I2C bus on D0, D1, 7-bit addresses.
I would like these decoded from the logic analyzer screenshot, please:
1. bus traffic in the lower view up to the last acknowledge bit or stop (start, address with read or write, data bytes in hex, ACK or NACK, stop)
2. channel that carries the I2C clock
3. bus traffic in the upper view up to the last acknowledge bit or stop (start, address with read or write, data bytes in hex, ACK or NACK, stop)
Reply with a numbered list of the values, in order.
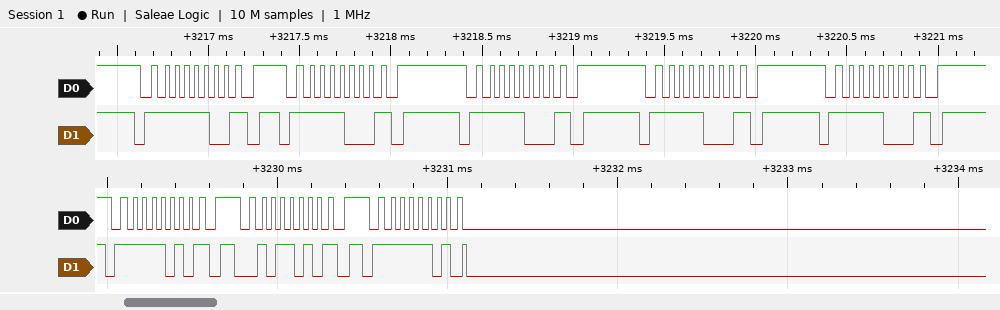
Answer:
1. start, address 7D write NACK, stop, start, address 2D write NACK, stop, start, address 7E read ACK
2. D0
3. start, address 7E write NACK, stop, start, address 7C write NACK, stop, start, address 7C write NACK, stop, start, address 7C write NACK, stop, start, address 7C write NACK, stop
